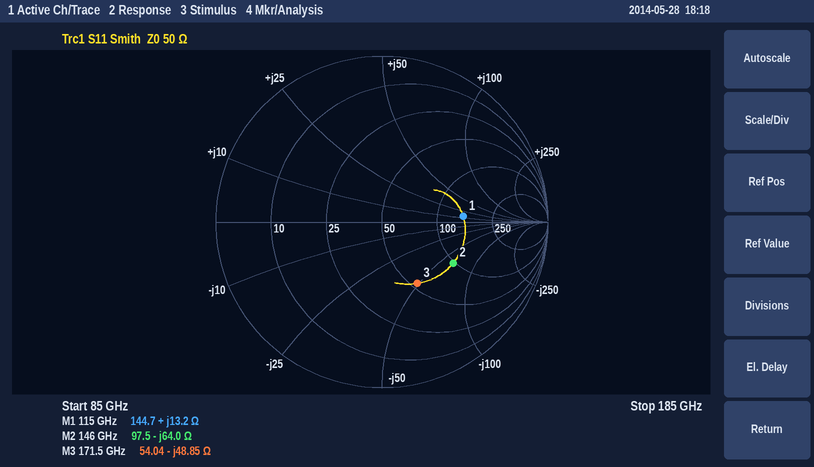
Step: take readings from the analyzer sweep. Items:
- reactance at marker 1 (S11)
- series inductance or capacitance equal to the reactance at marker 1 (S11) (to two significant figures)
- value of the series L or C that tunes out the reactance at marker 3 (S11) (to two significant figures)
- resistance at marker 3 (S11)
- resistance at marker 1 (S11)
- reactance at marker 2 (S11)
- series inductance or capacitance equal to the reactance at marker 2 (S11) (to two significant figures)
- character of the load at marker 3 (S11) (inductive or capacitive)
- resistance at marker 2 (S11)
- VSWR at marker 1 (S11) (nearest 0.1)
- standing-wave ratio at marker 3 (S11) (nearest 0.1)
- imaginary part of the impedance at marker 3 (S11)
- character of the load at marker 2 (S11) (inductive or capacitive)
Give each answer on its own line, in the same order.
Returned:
+13.2 Ω
18 pH
45 pH
54.04 Ω
144.7 Ω
-64.0 Ω
17 fF
capacitive
97.5 Ω
2.9
2.5
-48.85 Ω
capacitive
